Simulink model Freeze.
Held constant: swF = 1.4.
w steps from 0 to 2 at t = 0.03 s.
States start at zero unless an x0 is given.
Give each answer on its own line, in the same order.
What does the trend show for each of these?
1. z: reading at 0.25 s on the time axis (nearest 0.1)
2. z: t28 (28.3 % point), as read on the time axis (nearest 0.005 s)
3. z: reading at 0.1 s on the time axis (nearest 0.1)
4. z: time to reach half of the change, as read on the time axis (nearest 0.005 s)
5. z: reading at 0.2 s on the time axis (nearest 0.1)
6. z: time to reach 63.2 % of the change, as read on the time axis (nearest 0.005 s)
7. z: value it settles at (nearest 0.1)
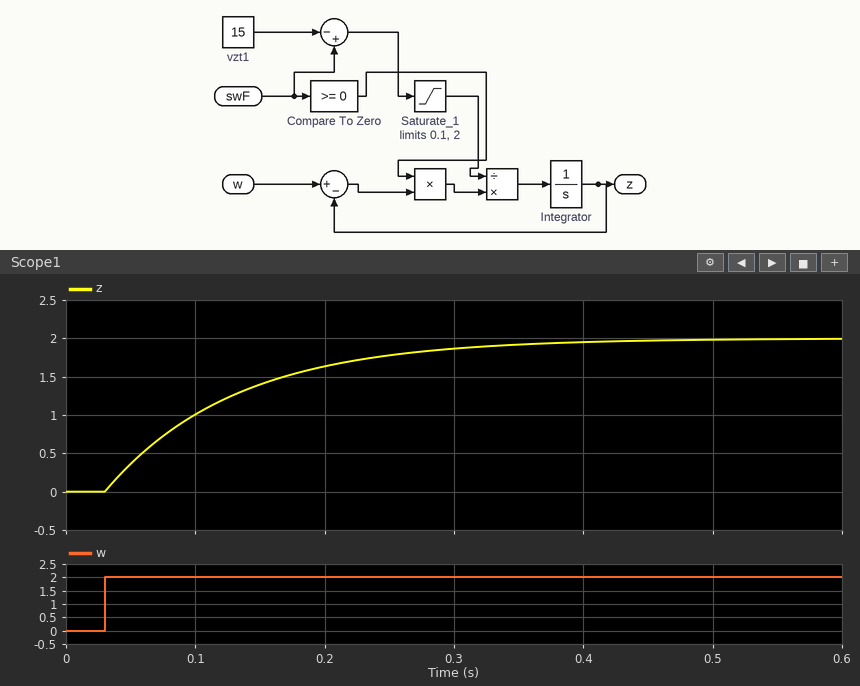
1.8
0.065 s
1.0
0.100 s
1.6
0.130 s
2.0
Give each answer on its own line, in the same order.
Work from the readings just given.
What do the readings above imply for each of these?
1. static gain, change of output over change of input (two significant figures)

1.0
